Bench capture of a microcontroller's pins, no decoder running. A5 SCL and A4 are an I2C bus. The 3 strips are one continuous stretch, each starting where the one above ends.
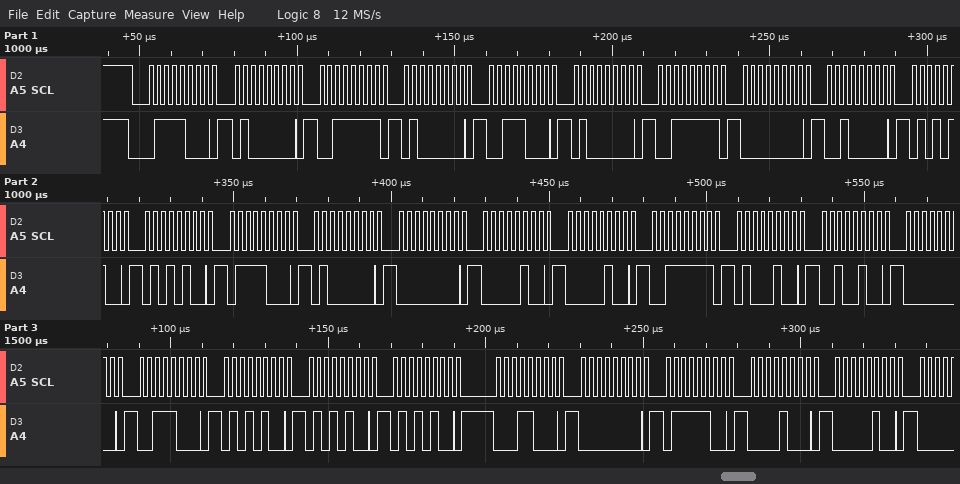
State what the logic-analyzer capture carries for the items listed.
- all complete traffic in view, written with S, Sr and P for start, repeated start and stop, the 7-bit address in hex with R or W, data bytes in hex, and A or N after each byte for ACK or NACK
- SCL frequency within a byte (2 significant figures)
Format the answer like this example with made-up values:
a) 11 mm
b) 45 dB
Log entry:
a) S 3CW A 40 A 3F A 40 A 38 A 40 A 3F A 00 A 20 A 54 A 54 A 78 A 40 A 00 A 04 A 04 A 3F A 44 A 24 A 00 A 38 A 54 A 54 A 54 A 18 A 00 A 7C A 08 A 04 A
b) 400 kHz
